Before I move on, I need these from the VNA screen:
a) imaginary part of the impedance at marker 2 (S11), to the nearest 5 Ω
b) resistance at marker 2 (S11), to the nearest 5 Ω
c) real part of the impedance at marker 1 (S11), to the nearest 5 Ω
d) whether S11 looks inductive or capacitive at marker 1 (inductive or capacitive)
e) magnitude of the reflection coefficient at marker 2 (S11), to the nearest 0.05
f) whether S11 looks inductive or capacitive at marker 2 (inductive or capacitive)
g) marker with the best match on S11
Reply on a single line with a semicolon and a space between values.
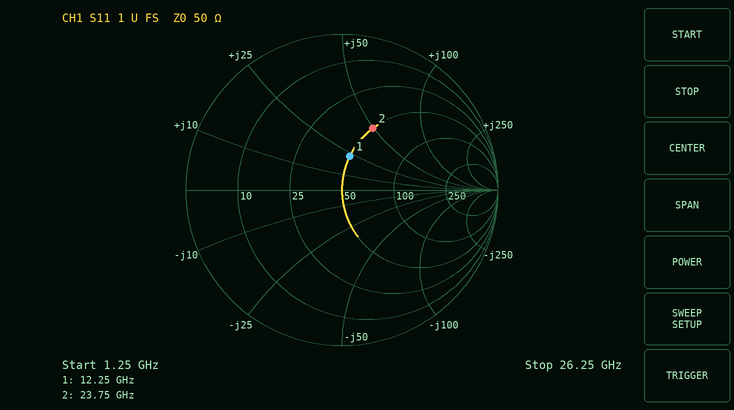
+50 Ω; 50 Ω; 50 Ω; inductive; 0.45; inductive; marker 1
